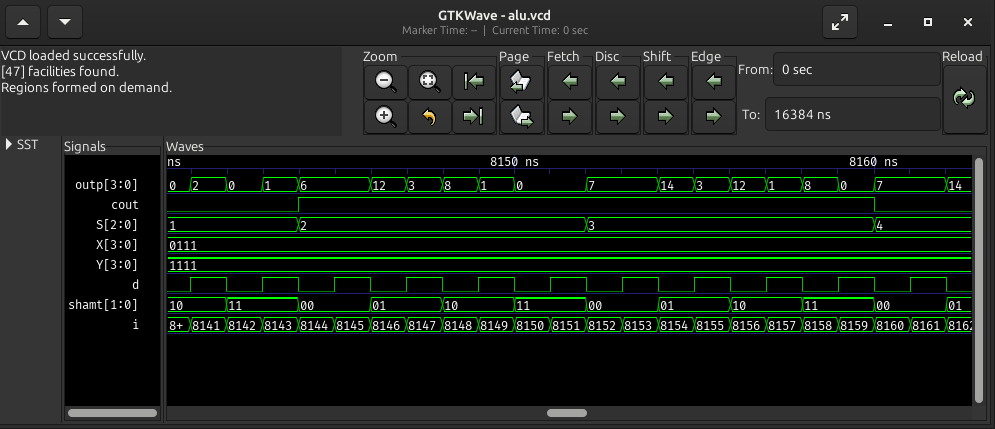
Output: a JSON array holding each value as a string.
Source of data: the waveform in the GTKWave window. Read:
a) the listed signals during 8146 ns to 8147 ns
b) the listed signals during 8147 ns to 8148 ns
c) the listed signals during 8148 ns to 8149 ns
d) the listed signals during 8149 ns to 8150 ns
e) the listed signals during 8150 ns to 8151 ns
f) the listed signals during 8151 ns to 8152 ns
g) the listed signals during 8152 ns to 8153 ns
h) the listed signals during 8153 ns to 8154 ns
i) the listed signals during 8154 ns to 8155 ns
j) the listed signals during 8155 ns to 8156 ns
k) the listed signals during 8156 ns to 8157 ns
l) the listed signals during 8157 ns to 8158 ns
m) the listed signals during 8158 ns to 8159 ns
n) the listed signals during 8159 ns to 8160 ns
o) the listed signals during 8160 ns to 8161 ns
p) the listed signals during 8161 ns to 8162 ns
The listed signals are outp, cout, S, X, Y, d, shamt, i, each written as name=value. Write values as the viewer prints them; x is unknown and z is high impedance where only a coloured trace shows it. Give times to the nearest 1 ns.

["outp=12, cout=1, S=2, X=0111, Y=1111, d=0, shamt=01, i=8146", "outp=3, cout=1, S=2, X=0111, Y=1111, d=1, shamt=01, i=8147", "outp=8, cout=1, S=2, X=0111, Y=1111, d=0, shamt=10, i=8148", "outp=1, cout=1, S=2, X=0111, Y=1111, d=1, shamt=10, i=8149", "outp=0, cout=1, S=2, X=0111, Y=1111, d=0, shamt=11, i=8150", "outp=0, cout=1, S=2, X=0111, Y=1111, d=1, shamt=11, i=8151", "outp=7, cout=1, S=3, X=0111, Y=1111, d=0, shamt=00, i=8152", "outp=7, cout=1, S=3, X=0111, Y=1111, d=1, shamt=00, i=8153", "outp=14, cout=1, S=3, X=0111, Y=1111, d=0, shamt=01, i=8154", "outp=3, cout=1, S=3, X=0111, Y=1111, d=1, shamt=01, i=8155", "outp=12, cout=1, S=3, X=0111, Y=1111, d=0, shamt=10, i=8156", "outp=1, cout=1, S=3, X=0111, Y=1111, d=1, shamt=10, i=8157", "outp=8, cout=1, S=3, X=0111, Y=1111, d=0, shamt=11, i=8158", "outp=0, cout=1, S=3, X=0111, Y=1111, d=1, shamt=11, i=8159", "outp=7, cout=0, S=4, X=0111, Y=1111, d=0, shamt=00, i=8160", "outp=7, cout=0, S=4, X=0111, Y=1111, d=1, shamt=00, i=8161"]
